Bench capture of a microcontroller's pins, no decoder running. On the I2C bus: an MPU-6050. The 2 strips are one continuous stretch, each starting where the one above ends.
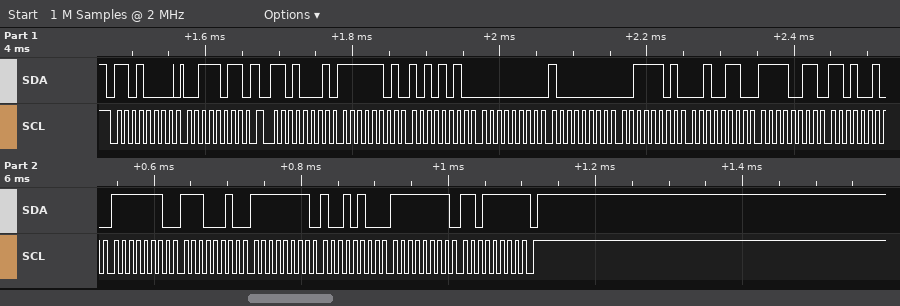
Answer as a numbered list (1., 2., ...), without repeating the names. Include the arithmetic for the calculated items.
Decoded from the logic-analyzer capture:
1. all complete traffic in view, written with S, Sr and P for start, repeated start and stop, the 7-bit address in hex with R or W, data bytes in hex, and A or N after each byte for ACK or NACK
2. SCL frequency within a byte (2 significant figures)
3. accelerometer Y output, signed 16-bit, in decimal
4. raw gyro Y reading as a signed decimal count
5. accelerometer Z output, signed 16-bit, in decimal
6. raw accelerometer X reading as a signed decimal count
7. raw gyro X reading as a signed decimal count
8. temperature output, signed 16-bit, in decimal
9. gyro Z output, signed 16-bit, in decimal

1. S 68W A 3B A Sr 68R A FD A AA A 00 A 80 A 3D A 26 A F3 A D2 A FE A E2 A FF A 94 A FF A DF N P
2. 100 kHz
3. 0x0080 = 128
4. 0xFF94 = -108
5. 0x3D26 = 15654
6. 0xFDAA = -598
7. 0xFEE2 = -286
8. 0xF3D2 = -3118
9. 0xFFDF = -33
